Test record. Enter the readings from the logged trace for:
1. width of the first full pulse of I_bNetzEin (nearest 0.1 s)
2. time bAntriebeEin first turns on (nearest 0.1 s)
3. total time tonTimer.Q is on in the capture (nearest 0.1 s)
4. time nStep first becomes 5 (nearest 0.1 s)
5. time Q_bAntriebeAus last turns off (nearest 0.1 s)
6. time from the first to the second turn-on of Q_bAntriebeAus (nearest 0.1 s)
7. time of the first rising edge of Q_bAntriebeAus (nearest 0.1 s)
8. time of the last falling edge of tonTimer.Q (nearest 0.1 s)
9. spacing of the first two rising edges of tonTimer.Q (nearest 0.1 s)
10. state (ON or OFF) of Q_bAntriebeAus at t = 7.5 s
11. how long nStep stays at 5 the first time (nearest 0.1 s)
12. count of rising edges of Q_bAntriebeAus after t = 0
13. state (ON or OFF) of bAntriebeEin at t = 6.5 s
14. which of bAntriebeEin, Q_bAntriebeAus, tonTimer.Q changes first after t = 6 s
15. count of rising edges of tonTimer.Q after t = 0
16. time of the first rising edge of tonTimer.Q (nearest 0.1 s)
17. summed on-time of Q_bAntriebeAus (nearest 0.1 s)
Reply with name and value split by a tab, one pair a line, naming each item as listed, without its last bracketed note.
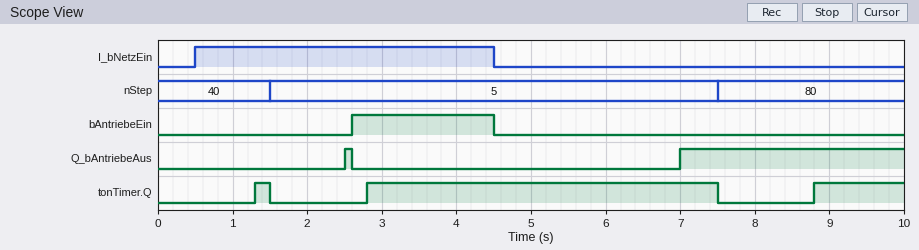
width of the first full pulse of I_bNetzEin	4.0 s
time bAntriebeEin first turns on	2.6 s
total time tonTimer.Q is on in the capture	6.1 s
time nStep first becomes 5	1.5 s
time Q_bAntriebeAus last turns off	2.6 s
time from the first to the second turn-on of Q_bAntriebeAus	4.5 s
time of the first rising edge of Q_bAntriebeAus	2.5 s
time of the last falling edge of tonTimer.Q	7.5 s
spacing of the first two rising edges of tonTimer.Q	1.5 s
state (ON or OFF) of Q_bAntriebeAus at t = 7.5 s	ON
how long nStep stays at 5 the first time	6.0 s
count of rising edges of Q_bAntriebeAus after t = 0	2
state (ON or OFF) of bAntriebeEin at t = 6.5 s	OFF
which of bAntriebeEin, Q_bAntriebeAus, tonTimer.Q changes first after t = 6 s	Q_bAntriebeAus
count of rising edges of tonTimer.Q after t = 0	3
time of the first rising edge of tonTimer.Q	1.3 s
summed on-time of Q_bAntriebeAus	3.1 s
